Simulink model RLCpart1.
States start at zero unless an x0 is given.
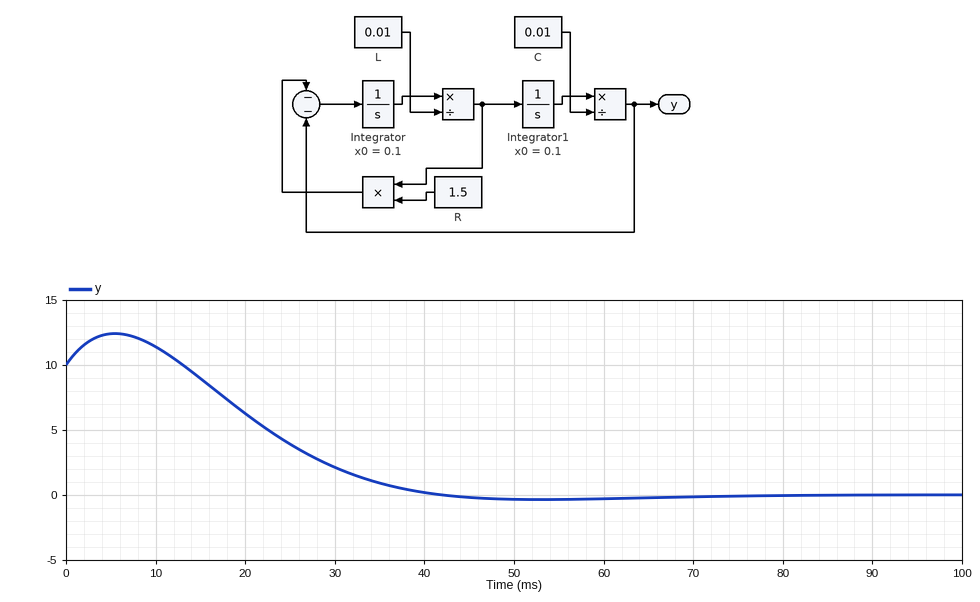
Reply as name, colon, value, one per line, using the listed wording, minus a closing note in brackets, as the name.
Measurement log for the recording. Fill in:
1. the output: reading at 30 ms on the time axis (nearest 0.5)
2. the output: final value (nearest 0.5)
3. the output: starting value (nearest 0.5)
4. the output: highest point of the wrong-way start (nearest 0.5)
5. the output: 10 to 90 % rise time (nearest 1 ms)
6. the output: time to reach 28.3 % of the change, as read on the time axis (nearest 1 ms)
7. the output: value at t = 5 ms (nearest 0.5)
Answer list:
the output: reading at 30 ms on the time axis: 2.0
the output: final value: 0.0
the output: starting value: 10.0
the output: highest point of the wrong-way start: 12.5
the output: 10 to 90 % rise time: 20 ms
the output: time to reach 28.3 % of the change, as read on the time axis: 18 ms
the output: value at t = 5 ms: 12.5
